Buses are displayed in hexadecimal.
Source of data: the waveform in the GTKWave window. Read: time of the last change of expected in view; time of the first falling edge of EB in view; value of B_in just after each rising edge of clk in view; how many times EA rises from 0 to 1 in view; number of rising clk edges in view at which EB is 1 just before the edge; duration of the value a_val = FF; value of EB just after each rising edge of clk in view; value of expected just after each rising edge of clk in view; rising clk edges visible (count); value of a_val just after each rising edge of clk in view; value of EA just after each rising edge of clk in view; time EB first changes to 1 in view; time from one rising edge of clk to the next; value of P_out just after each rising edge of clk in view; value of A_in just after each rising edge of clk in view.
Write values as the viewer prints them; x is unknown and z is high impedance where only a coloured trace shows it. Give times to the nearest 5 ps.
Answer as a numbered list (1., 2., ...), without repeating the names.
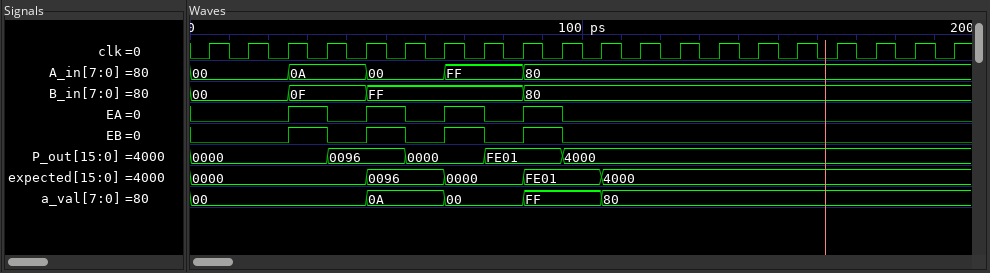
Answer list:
1. 105 ps
2. 35 ps
3. 00, 00, 0F, 0F, FF, FF, FF, FF, 80, 80, 80, 80, 80, 80, 80, 80, 80, 80, 80, 80
4. 4
5. 4
6. 20 ps
7. 0 0 1 0 1 0 1 0 1 0 0 0 0 0 0 0 0 0 0 0
8. 0000, 0000, 0000, 0000, 0096, 0096, 0000, 0000, FE01, FE01, 4000, 4000, 4000, 4000, 4000, 4000, 4000, 4000, 4000, 4000
9. 20
10. 00, 00, 00, 00, 0A, 0A, 00, 00, FF, FF, 80, 80, 80, 80, 80, 80, 80, 80, 80, 80
11. 0 0 1 0 1 0 1 0 1 0 0 0 0 0 0 0 0 0 0 0
12. 25 ps
13. 10 ps
14. 0000, 0000, 0000, 0096, 0096, 0000, 0000, FE01, FE01, 4000, 4000, 4000, 4000, 4000, 4000, 4000, 4000, 4000, 4000, 4000
15. 00, 00, 0A, 0A, 00, 00, FF, FF, 80, 80, 80, 80, 80, 80, 80, 80, 80, 80, 80, 80
